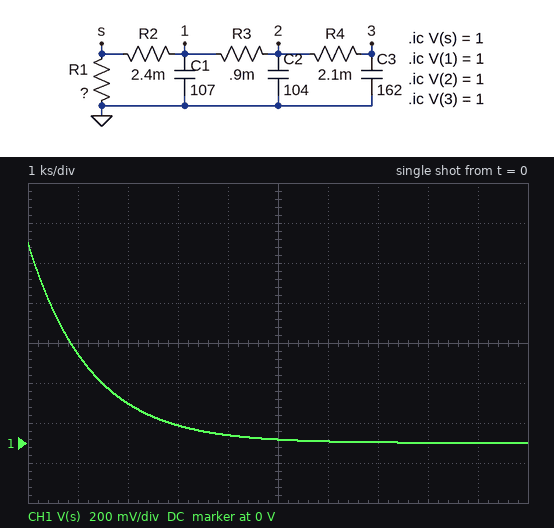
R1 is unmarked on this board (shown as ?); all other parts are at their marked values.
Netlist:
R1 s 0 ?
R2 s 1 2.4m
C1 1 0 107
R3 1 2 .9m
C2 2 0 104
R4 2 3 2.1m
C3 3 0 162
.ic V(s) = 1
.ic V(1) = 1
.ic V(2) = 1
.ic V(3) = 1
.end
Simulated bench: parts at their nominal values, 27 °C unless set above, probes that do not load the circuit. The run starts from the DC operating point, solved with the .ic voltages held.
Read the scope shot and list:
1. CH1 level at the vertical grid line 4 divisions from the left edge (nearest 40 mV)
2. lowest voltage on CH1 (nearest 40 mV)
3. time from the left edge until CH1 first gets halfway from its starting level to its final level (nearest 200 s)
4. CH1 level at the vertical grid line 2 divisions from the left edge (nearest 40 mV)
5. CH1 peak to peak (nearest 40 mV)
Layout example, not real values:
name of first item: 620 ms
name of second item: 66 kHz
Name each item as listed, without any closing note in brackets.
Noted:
CH1 level at the vertical grid line 4 divisions from the left edge: 40 mV
lowest voltage on CH1: 0 V
time from the left edge until CH1 first gets halfway from its starting level to its final level: 800 s
CH1 level at the vertical grid line 2 divisions from the left edge: 200 mV
CH1 peak to peak: 1.00 V
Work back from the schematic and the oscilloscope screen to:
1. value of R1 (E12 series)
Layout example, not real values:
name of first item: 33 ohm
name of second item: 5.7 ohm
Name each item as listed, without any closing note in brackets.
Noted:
value of R1: 3.3 Ω
